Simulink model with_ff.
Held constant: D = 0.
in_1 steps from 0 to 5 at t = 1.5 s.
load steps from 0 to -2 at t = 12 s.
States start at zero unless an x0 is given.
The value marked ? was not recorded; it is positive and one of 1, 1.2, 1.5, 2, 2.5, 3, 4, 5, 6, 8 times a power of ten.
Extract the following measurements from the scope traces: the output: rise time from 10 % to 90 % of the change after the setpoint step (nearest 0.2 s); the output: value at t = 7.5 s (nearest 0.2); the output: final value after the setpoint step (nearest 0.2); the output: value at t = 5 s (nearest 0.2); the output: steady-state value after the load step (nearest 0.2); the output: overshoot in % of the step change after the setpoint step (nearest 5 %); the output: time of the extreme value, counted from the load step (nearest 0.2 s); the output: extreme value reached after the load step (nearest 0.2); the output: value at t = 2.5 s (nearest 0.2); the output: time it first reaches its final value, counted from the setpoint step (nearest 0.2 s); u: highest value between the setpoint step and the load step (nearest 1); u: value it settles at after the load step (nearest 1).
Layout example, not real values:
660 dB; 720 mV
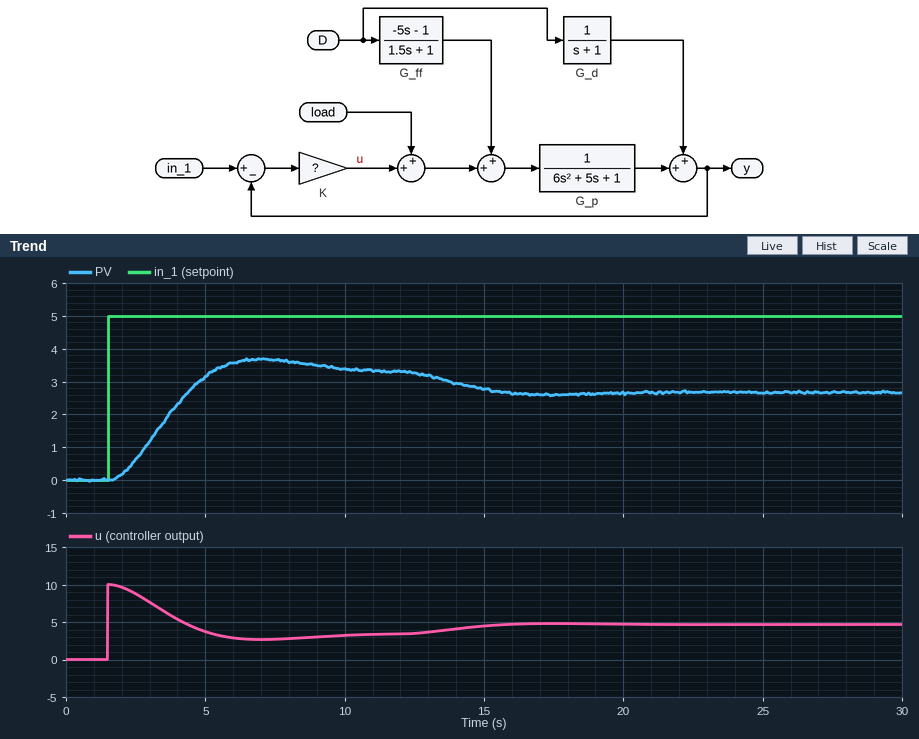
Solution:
2.6 s; 3.6; 3.4; 3.2; 2.6; 10 %; 5.4 s; 2.6; 0.6; 3.8 s; 10; 5
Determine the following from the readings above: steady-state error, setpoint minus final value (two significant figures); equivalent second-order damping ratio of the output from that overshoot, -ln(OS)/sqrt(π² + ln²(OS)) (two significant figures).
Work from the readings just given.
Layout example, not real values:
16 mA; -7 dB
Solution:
1.6; 0.59
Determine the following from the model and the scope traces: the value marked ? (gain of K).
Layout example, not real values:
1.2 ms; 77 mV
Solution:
2
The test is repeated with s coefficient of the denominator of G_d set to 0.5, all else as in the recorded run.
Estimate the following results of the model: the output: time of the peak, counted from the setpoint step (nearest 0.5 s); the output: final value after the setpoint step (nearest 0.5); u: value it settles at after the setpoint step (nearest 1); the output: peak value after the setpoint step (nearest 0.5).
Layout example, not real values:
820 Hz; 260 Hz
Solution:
5.5 s; 3.5; 3; 3.5
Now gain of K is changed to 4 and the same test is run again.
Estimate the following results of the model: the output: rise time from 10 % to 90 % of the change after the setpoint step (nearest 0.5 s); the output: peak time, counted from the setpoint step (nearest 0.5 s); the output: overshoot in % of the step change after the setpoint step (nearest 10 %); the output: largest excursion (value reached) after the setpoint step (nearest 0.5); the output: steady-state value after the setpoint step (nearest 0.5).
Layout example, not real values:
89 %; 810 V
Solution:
1.5 s; 4.0 s; 20 %; 5.0; 4.0
